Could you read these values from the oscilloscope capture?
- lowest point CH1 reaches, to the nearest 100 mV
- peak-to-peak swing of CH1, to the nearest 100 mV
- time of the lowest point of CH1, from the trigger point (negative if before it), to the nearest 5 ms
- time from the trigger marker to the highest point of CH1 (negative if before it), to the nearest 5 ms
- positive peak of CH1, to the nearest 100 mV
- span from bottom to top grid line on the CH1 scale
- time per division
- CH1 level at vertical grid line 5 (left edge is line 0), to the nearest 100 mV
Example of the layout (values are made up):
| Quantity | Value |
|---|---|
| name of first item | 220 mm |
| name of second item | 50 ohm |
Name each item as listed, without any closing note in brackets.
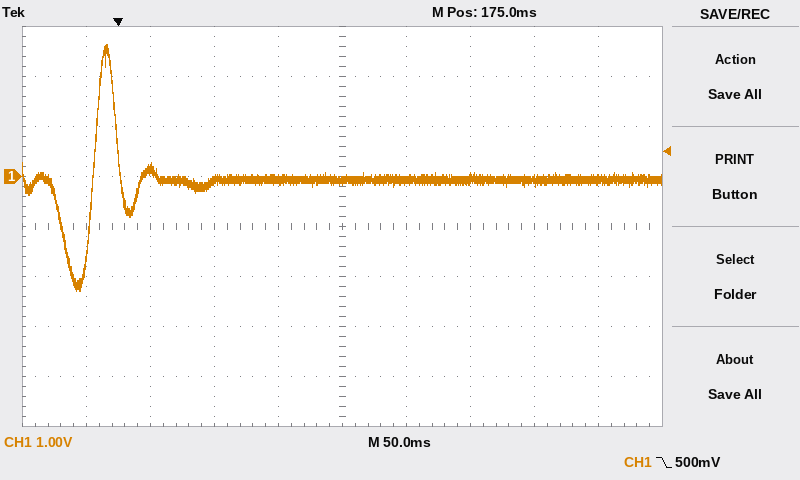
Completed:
| Quantity | Value |
|---|---|
| lowest point CH1 reaches, to the nearest 100 mV | -2.3 V |
| peak-to-peak swing of CH1, to the nearest 100 mV | 4.9 V |
| time of the lowest point of CH1, from the trigger point (negative if before it), to the nearest 5 ms | -30 ms |
| time from the trigger marker to the highest point of CH1 (negative if before it), to the nearest 5 ms | -10 ms |
| positive peak of CH1, to the nearest 100 mV | 2.6 V |
| span from bottom to top grid line on the CH1 scale | 8 V |
| time per division | 50 ms |
| CH1 level at vertical grid line 5 (left edge is line 0), to the nearest 100 mV | -100 mV |
